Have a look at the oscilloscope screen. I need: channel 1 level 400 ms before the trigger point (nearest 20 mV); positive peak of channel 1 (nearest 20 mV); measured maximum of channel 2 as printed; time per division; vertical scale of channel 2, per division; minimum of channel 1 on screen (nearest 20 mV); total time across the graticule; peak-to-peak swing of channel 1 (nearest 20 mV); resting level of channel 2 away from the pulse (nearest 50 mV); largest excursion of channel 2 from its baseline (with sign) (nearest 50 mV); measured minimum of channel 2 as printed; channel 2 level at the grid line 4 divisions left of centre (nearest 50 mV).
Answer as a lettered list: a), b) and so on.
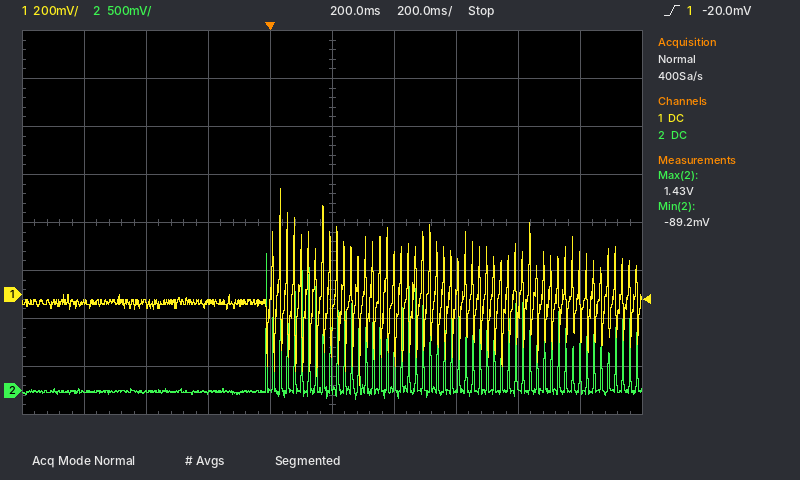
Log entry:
a) -40 mV
b) 440 mV
c) 1.43 V
d) 200 ms
e) 500 mV
f) -380 mV
g) 2 s
h) 820 mV
i) 0 mV
j) +1.45 V
k) -89.2 mV
l) 0 mV
